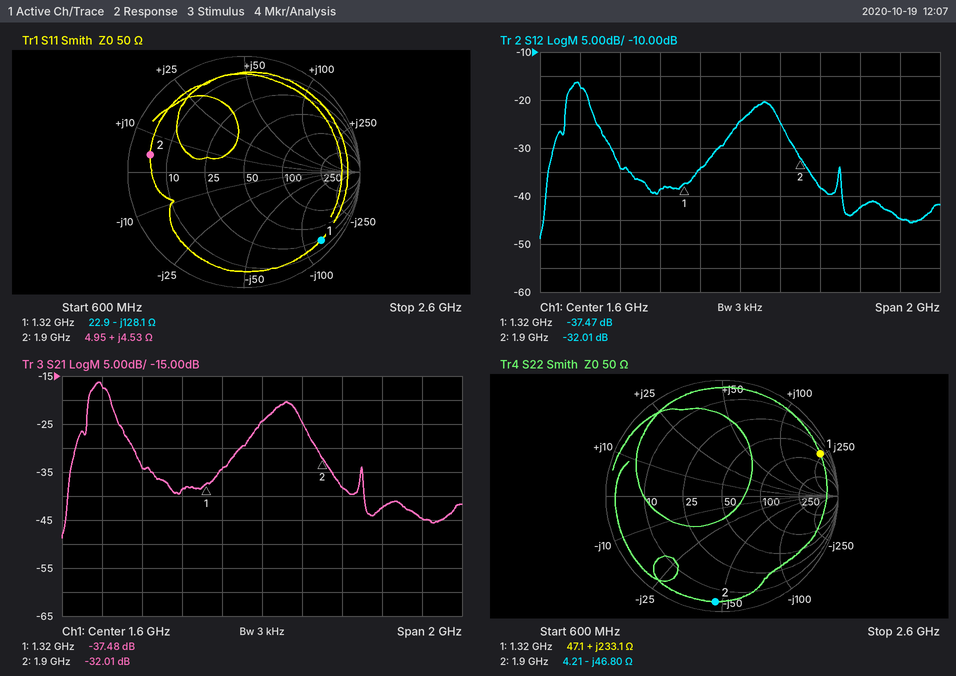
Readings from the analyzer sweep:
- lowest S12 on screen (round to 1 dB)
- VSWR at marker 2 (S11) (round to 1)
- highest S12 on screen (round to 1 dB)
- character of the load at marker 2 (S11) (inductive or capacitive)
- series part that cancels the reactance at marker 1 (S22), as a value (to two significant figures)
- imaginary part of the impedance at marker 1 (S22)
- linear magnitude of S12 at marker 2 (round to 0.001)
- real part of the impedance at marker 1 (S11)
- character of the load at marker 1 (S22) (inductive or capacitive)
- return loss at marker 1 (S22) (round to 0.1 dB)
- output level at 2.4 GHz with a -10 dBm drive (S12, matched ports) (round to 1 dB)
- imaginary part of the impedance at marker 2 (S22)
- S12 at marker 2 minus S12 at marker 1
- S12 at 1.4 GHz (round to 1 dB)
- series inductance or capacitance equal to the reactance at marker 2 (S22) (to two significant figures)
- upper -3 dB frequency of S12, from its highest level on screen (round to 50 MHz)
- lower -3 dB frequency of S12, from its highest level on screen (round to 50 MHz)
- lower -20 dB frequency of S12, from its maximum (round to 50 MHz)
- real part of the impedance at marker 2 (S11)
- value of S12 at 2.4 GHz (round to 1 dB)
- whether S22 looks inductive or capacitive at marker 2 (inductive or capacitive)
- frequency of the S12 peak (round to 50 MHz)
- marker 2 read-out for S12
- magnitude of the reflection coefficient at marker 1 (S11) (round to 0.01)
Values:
-49 dB
10
-16 dB
inductive
520 fF
+233.1 Ω
0.025
22.9 Ω
inductive
0.7 dB
-55 dBm
-46.80 Ω
5.46 dB
-34 dB
1.8 pF
850 MHz
750 MHz
650 MHz
4.95 Ω
-45 dB
capacitive
800 MHz
-32.01 dB
0.89
